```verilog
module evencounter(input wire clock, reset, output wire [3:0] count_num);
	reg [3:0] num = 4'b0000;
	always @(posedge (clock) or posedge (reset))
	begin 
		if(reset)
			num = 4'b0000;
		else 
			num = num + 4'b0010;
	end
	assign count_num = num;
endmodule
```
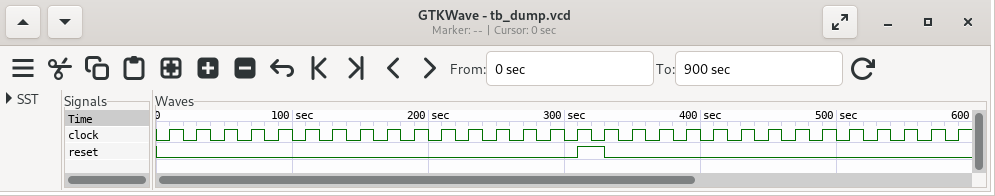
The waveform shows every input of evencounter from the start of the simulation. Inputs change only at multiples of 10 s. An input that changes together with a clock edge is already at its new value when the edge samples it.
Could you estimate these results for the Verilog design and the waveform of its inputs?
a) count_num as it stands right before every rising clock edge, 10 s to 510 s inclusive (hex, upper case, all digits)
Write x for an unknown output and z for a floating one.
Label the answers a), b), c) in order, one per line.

a) 0, 2, 4, 6, 8, A, C, E, 0, 2, 4, 6, 8, A, C, E, 0, 2, 4, 6, 8, A, C, E, 0, 2
